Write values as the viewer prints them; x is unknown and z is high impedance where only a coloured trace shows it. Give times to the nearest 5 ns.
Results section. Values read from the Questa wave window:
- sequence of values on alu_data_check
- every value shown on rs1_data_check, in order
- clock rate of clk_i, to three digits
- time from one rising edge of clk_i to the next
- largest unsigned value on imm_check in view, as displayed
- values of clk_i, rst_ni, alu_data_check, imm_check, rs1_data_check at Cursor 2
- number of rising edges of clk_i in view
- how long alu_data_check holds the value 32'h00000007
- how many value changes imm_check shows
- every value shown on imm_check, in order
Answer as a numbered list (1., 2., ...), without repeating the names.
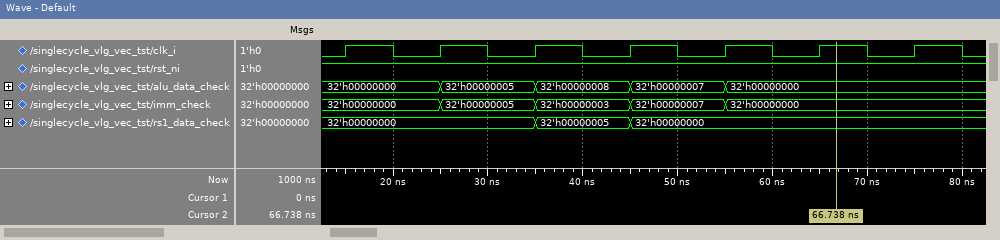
1. 32'h00000000, 32'h00000005, 32'h00000008, 32'h00000007, 32'h00000000
2. 32'h00000000, 32'h00000005, 32'h00000000
3. 100 MHz
4. 10 ns
5. 32'h00000007
6. clk_i=1, rst_ni=1, alu_data_check=32'h00000000, imm_check=32'h00000000, rs1_data_check=32'h00000000
7. 7
8. 10 ns
9. 4
10. 32'h00000000, 32'h00000005, 32'h00000003, 32'h00000007, 32'h00000000
